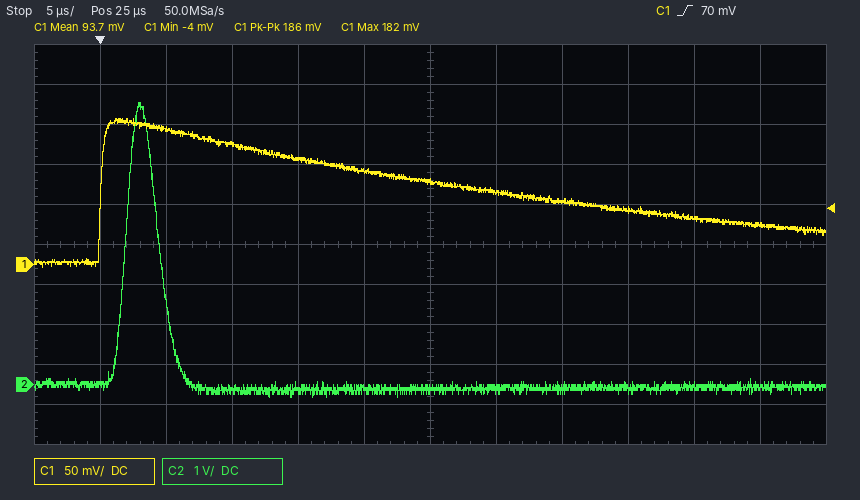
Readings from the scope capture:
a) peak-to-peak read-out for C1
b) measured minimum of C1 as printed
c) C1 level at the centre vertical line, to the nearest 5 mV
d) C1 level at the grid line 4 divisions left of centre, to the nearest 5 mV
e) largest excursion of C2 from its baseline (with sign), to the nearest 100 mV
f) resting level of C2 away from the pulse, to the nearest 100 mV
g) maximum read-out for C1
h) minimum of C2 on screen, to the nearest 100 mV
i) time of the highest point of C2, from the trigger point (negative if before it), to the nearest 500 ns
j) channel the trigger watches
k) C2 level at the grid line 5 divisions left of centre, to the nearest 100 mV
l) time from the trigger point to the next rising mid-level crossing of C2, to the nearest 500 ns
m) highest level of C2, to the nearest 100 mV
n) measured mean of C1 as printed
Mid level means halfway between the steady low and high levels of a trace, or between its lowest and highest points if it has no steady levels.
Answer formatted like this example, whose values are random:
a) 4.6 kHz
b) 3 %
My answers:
a) 186 mV
b) -4 mV
c) 105 mV
d) 170 mV
e) +7.1 V
f) -100 mV
g) 182 mV
h) -300 mV
i) +3.0 µs
j) C1
k) 0.0 V
l) 2.0 µs
m) 7.0 V
n) 93.7 mV
